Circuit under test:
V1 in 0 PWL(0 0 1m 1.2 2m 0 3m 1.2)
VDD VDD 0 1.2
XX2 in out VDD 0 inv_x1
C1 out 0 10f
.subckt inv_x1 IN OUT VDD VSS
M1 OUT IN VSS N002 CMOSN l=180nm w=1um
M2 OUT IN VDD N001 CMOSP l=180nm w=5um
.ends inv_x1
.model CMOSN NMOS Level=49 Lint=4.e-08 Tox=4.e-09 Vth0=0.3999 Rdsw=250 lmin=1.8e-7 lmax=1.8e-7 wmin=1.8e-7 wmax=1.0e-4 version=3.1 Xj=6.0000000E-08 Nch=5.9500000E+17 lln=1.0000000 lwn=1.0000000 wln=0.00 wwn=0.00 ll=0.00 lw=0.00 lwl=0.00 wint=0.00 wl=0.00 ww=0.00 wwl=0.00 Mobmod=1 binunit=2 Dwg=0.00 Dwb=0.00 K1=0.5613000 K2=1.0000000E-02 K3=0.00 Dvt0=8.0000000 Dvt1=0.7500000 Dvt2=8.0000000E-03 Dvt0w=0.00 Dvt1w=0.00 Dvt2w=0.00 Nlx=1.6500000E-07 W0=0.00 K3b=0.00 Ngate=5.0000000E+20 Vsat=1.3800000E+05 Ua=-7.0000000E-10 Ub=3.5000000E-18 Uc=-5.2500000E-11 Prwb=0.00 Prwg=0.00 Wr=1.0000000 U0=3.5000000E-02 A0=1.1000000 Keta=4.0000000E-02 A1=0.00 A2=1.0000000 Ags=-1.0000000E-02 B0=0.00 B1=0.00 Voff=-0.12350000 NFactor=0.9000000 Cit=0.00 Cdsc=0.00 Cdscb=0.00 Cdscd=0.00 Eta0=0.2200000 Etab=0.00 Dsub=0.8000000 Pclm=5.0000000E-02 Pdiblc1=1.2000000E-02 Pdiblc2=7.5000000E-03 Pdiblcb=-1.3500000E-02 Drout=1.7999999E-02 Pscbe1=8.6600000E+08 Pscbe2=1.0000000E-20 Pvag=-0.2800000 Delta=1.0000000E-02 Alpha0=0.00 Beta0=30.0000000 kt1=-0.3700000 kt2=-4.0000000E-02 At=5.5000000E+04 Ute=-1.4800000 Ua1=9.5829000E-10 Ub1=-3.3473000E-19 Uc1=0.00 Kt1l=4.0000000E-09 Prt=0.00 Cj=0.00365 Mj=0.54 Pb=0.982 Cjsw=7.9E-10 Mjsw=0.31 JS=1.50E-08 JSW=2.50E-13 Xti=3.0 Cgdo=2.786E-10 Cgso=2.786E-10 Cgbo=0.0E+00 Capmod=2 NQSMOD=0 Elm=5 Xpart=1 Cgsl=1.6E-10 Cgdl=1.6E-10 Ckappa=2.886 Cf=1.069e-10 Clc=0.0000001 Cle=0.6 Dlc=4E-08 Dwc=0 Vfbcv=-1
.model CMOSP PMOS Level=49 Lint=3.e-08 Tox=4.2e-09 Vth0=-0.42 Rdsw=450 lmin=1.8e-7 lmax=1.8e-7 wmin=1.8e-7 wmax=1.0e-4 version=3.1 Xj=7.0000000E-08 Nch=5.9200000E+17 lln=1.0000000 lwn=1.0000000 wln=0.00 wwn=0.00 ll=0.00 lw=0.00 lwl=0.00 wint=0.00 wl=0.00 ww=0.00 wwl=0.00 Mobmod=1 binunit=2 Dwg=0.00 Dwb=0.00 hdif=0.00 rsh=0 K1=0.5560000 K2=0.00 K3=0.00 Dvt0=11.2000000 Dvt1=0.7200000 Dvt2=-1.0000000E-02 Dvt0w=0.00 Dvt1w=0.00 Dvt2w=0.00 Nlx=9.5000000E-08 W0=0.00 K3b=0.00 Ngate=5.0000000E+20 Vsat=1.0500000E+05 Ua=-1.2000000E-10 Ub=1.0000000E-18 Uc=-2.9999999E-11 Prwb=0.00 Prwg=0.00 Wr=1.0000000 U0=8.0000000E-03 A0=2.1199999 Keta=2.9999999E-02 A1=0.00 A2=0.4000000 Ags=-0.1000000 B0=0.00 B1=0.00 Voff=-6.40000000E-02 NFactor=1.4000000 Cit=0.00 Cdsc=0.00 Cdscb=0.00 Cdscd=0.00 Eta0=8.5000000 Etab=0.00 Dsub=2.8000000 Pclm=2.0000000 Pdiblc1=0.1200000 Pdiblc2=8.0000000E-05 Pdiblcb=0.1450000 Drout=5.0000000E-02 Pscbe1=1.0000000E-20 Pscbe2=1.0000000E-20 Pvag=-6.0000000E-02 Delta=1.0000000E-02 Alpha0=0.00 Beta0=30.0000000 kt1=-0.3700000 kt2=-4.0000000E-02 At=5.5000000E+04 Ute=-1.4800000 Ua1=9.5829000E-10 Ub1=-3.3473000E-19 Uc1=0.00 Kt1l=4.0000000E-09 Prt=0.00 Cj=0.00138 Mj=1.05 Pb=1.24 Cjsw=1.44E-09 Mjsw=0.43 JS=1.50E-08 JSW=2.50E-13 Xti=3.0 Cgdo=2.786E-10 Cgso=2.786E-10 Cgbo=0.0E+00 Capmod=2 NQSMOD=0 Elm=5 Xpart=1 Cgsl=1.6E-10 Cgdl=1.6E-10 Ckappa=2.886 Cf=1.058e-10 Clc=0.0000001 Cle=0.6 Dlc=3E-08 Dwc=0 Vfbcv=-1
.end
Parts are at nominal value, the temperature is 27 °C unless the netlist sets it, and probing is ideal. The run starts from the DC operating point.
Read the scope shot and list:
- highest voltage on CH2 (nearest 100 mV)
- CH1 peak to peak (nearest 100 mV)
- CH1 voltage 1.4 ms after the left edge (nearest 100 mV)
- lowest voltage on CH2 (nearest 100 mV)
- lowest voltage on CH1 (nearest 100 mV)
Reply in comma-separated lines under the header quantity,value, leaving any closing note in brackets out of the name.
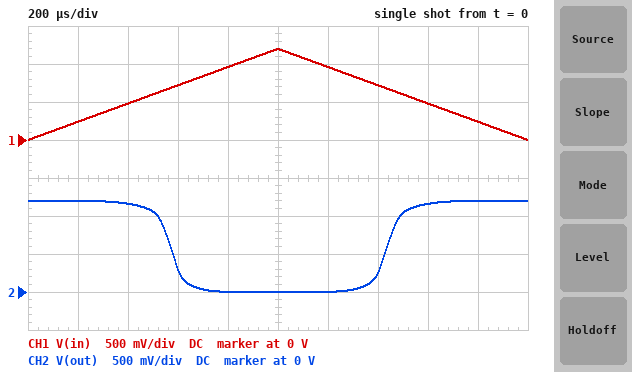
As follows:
quantity,value
highest voltage on CH2,1.2 V
CH1 peak to peak,1.2 V
CH1 voltage 1.4 ms after the left edge,700 mV
lowest voltage on CH2,0 V
lowest voltage on CH1,0 V
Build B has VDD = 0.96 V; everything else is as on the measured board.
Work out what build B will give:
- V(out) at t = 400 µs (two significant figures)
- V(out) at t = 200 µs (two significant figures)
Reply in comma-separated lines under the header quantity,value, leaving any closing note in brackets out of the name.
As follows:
quantity,value
V(out) at t = 400 µs,880 mV
V(out) at t = 200 µs,960 mV
